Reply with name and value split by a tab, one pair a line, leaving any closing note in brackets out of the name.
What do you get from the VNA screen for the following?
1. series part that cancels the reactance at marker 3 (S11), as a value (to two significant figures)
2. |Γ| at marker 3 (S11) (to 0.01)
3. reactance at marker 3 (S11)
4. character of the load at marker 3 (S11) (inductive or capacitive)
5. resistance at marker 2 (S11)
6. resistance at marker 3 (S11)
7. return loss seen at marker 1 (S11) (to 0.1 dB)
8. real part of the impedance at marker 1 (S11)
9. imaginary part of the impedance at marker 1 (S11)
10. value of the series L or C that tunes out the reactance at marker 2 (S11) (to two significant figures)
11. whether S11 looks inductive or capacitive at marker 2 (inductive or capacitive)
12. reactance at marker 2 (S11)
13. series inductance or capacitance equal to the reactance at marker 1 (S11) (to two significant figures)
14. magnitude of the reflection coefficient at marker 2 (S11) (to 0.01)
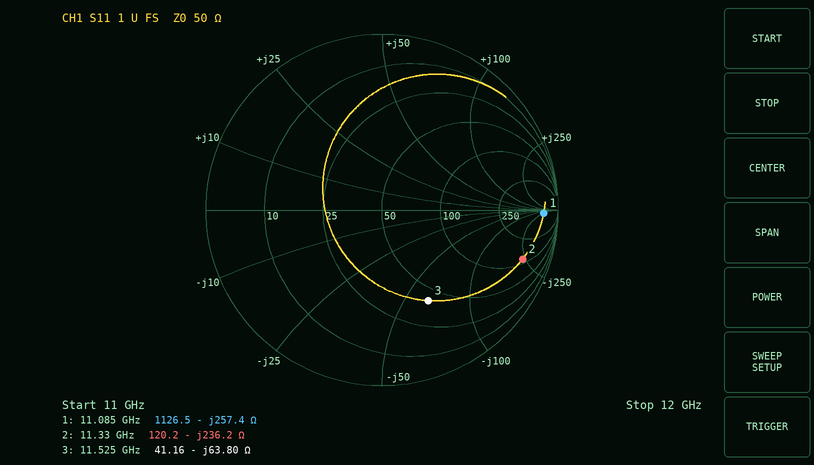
series part that cancels the reactance at marker 3 (S11), as a value	880 pH
|Γ| at marker 3 (S11)	0.58
reactance at marker 3	-63.80 Ω
character of the load at marker 3 (S11)	capacitive
resistance at marker 2	120.2 Ω
resistance at marker 3	41.16 Ω
return loss seen at marker 1 (S11)	0.7 dB
real part of the impedance at marker 1	1126.5 Ω
imaginary part of the impedance at marker 1	-257.4 Ω
value of the series L or C that tunes out the reactance at marker 2 (S11)	3.3 nH
whether S11 looks inductive or capacitive at marker 2	capacitive
reactance at marker 2	-236.2 Ω
series inductance or capacitance equal to the reactance at marker 1 (S11)	56 fF
magnitude of the reflection coefficient at marker 2 (S11)	0.85
